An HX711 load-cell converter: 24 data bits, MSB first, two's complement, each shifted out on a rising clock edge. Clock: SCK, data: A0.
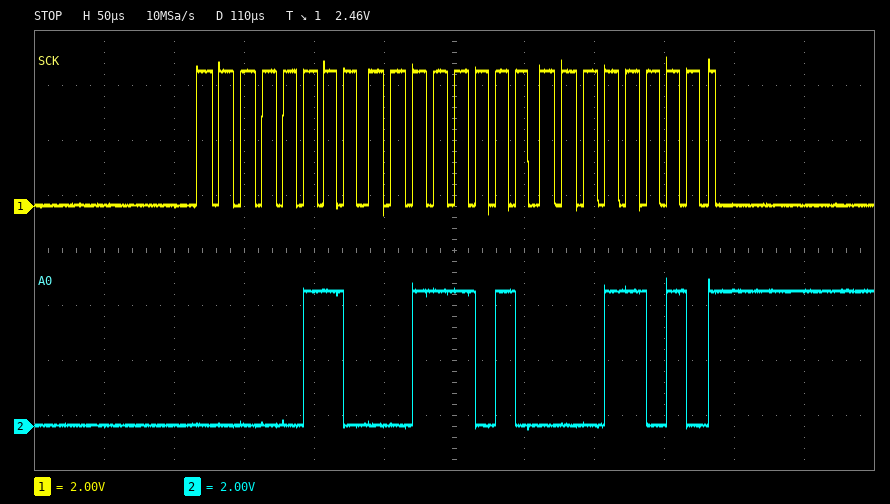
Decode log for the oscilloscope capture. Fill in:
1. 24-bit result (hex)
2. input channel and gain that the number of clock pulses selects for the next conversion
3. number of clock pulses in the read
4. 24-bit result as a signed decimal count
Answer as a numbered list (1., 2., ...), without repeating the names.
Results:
1. 0x063A1A
2. channel A, gain 128
3. 25
4. 408090
